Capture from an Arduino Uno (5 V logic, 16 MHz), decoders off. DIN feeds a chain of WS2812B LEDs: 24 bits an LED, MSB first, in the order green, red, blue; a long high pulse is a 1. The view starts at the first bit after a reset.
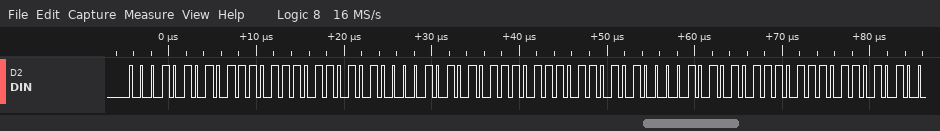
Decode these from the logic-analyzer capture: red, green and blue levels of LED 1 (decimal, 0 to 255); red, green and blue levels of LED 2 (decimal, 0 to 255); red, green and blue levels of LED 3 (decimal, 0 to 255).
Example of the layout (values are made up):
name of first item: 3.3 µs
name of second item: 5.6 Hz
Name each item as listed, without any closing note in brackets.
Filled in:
red, green and blue levels of LED 1: 119, 21, 106
red, green and blue levels of LED 2: 119, 21, 106
red, green and blue levels of LED 3: 119, 21, 106
